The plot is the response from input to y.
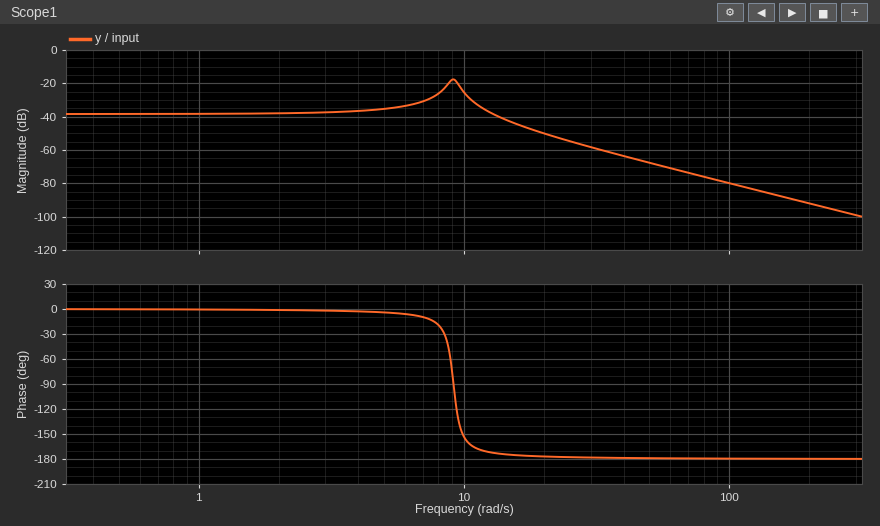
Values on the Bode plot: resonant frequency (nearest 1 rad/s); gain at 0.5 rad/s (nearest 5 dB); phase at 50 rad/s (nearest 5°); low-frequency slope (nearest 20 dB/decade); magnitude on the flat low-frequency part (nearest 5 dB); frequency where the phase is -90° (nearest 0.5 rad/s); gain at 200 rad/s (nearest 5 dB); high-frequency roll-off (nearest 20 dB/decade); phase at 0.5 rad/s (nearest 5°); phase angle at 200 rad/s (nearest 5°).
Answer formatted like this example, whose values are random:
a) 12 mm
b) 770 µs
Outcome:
a) 9 rad/s
b) -40 dB
c) -180°
d) 0 dB/decade
e) -40 dB
f) 9.0 rad/s
g) -90 dB
h) -40 dB/decade
i) 0°
j) -180°
